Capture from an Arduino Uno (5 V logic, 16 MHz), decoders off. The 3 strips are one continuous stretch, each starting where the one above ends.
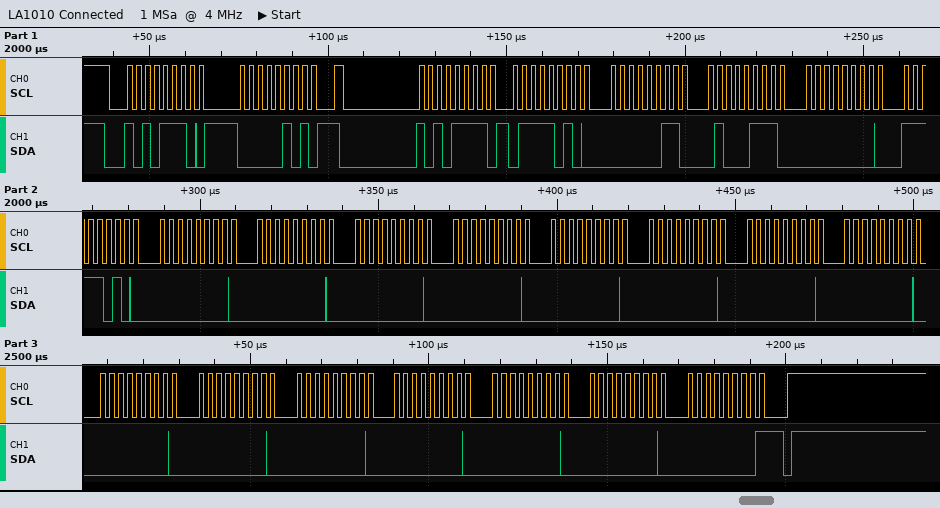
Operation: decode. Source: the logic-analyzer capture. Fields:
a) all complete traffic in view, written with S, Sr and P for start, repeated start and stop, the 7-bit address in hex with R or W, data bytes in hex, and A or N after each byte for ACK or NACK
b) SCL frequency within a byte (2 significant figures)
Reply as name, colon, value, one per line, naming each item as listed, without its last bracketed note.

all complete traffic in view, written with S, Sr and P for start, repeated start and stop, the 7-bit address in hex with R or W, data bytes in hex, and A or N after each byte for ACK or NACK: S 57W A 05 A Sr 57R A 7A A 03 A 47 A 00 A FA A 00 A 00 A 00 A 00 A 00 A 00 A 00 A 00 A 00 A 00 A 00 A 00 A 00 A 00 A 00 N P
SCL frequency within a byte: 400 kHz
